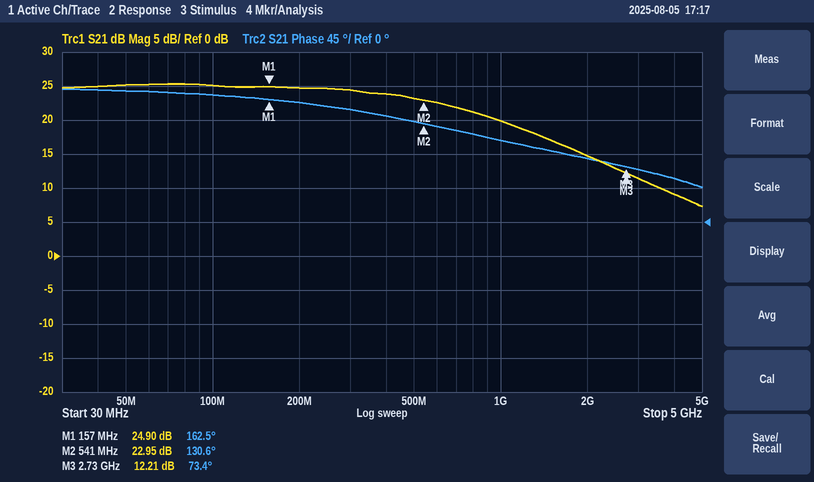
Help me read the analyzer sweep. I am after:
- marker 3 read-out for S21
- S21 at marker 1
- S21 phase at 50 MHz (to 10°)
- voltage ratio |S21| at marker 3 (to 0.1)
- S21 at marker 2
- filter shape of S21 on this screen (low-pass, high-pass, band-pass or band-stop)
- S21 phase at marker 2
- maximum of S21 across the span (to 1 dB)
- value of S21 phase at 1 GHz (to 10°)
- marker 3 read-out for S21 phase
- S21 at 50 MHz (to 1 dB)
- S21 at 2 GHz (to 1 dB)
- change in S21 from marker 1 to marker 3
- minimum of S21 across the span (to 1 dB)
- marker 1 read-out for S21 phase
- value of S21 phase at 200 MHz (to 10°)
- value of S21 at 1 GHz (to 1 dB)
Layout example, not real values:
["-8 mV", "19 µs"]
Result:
["12.21 dB", "24.90 dB", "170°", "4.1", "22.95 dB", "low-pass", "130.6°", "25 dB", "110°", "73.4°", "25 dB", "15 dB", "-12.69 dB", "7 dB", "162.5°", "160°", "20 dB"]
